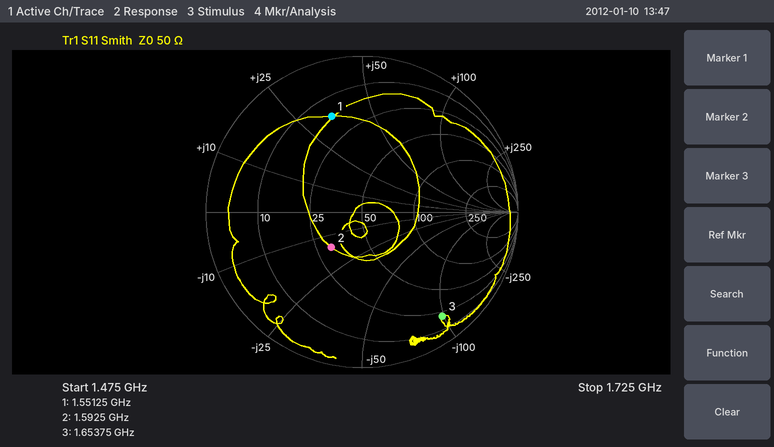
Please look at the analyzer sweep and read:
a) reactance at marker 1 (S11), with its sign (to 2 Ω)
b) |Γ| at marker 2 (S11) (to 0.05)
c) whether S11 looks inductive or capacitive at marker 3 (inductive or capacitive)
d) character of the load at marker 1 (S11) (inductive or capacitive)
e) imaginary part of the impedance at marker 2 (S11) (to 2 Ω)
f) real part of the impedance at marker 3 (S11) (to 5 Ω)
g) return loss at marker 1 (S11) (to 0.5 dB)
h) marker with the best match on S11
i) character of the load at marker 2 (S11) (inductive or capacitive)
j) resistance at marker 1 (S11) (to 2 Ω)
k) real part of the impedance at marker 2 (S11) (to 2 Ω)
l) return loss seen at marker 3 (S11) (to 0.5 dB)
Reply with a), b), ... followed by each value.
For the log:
a) +34 Ω
b) 0.30
c) capacitive
d) inductive
e) -16 Ω
f) 20 Ω
g) 4.0 dB
h) marker 2
i) capacitive
j) 16 Ω
k) 30 Ω
l) 1.5 dB
